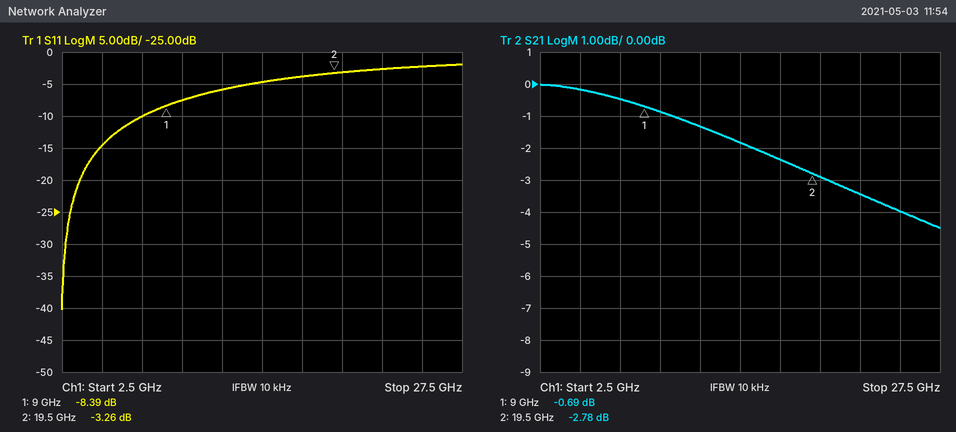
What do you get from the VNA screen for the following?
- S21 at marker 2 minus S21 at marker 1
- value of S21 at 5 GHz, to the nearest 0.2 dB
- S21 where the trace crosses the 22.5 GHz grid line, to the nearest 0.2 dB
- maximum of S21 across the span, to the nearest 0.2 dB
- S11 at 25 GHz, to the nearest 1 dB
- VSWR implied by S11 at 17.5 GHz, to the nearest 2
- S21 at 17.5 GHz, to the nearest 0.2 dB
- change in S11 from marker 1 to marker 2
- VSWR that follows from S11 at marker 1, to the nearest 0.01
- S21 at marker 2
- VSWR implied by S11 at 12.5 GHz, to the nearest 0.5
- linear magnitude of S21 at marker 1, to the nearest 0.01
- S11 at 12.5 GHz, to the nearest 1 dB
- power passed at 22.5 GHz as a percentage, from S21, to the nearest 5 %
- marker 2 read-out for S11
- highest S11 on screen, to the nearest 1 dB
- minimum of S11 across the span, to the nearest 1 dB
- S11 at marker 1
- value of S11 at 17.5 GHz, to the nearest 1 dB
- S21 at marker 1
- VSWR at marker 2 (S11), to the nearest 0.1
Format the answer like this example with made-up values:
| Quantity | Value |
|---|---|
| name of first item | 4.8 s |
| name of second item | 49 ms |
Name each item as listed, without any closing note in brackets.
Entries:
| Quantity | Value |
|---|---|
| S21 at marker 2 minus S21 at marker 1 | -2.09 dB |
| value of S21 at 5 GHz, to the nearest 0.2 dB | -0.2 dB |
| S21 where the trace crosses the 22.5 GHz grid line, to the nearest 0.2 dB | -3.4 dB |
| maximum of S21 across the span, to the nearest 0.2 dB | 0.0 dB |
| S11 at 25 GHz, to the nearest 1 dB | -2 dB |
| VSWR implied by S11 at 17.5 GHz, to the nearest 2 | 4 |
| S21 at 17.5 GHz, to the nearest 0.2 dB | -2.4 dB |
| change in S11 from marker 1 to marker 2 | 5.13 dB |
| VSWR that follows from S11 at marker 1, to the nearest 0.01 | 2.23 |
| S21 at marker 2 | -2.78 dB |
| VSWR implied by S11 at 12.5 GHz, to the nearest 0.5 | 3.0 |
| linear magnitude of S21 at marker 1, to the nearest 0.01 | 0.92 |
| S11 at 12.5 GHz, to the nearest 1 dB | -6 dB |
| power passed at 22.5 GHz as a percentage, from S21, to the nearest 5 % | 45 % |
| marker 2 read-out for S11 | -3.26 dB |
| highest S11 on screen, to the nearest 1 dB | -2 dB |
| minimum of S11 across the span, to the nearest 1 dB | -40 dB |
| S11 at marker 1 | -8.39 dB |
| value of S11 at 17.5 GHz, to the nearest 1 dB | -4 dB |
| S21 at marker 1 | -0.69 dB |
| VSWR at marker 2 (S11), to the nearest 0.1 | 5.4 |
